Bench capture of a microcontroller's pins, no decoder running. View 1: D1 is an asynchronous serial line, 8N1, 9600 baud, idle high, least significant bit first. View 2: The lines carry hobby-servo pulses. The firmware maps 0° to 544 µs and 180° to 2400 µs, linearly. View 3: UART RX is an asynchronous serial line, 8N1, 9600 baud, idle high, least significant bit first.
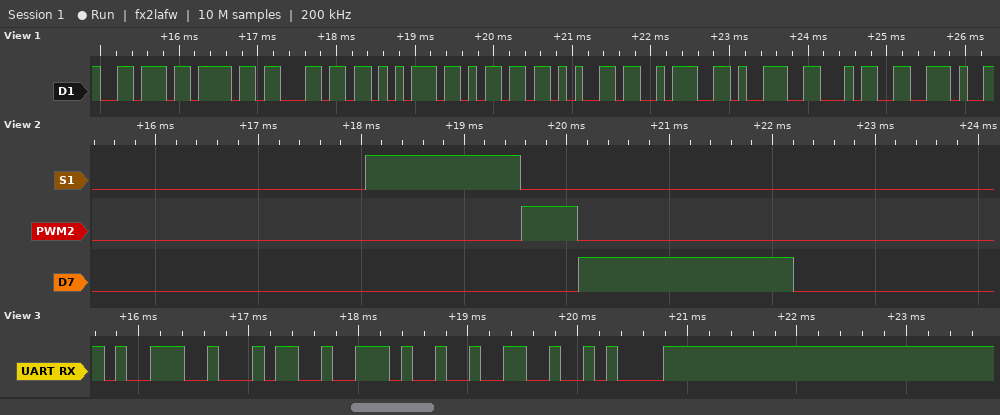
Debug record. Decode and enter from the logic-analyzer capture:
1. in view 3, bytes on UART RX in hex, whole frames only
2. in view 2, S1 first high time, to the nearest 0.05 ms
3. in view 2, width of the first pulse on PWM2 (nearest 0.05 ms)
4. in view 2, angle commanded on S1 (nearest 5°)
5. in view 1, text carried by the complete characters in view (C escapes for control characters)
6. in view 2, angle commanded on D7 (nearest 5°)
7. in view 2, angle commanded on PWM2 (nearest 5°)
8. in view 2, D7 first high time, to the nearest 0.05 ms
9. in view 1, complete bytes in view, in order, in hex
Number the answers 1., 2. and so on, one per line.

1. 39 34 2E 32 0A
2. 1.50 ms
3. 0.55 ms
4. 95°
5. "volume:94."
6. 150°
7. 0°
8. 2.10 ms
9. 76 6F 6C 75 6D 65 3A 39 34 2E
